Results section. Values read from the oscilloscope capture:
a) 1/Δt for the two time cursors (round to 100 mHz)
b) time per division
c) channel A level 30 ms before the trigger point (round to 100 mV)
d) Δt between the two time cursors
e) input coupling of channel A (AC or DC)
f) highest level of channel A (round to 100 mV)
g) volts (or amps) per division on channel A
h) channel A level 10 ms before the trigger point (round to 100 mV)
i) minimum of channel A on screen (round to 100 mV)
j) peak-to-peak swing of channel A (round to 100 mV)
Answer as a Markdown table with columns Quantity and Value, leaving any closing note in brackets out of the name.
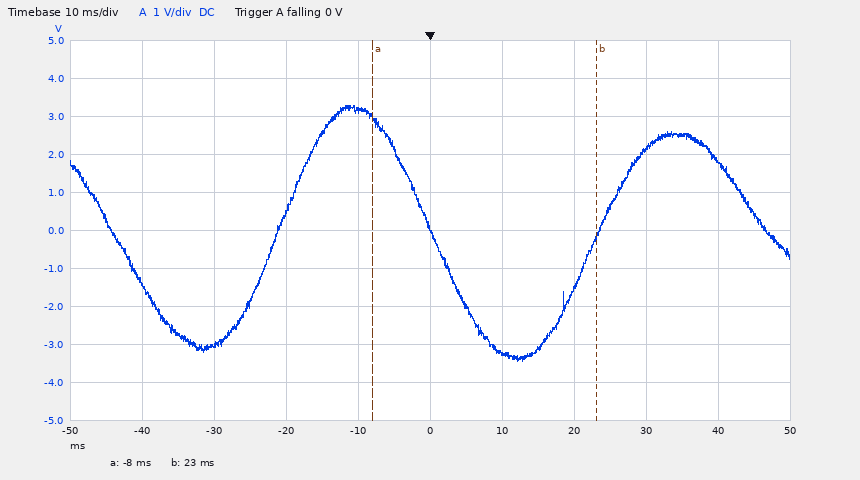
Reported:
| Quantity | Value |
|---|---|
| 1/Δt for the two time cursors | 32.3 Hz |
| time per division | 10 ms |
| channel A level 30 ms before the trigger point | -3.0 V |
| Δt between the two time cursors | 31 ms |
| input coupling of channel A | DC |
| highest level of channel A | 3.3 V |
| volts (or amps) per division on channel A | 1 V |
| channel A level 10 ms before the trigger point | 3.2 V |
| minimum of channel A on screen | -3.4 V |
| peak-to-peak swing of channel A | 6.7 V |
